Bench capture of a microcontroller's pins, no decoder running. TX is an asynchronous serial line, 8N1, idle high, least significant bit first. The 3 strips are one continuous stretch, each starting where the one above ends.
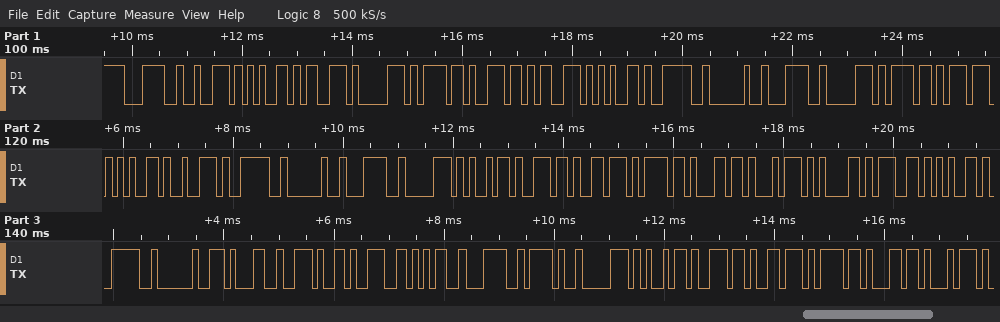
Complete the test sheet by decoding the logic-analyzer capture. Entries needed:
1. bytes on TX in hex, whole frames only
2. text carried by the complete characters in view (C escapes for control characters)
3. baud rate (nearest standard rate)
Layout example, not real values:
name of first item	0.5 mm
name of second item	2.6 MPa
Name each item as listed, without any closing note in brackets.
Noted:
bytes on TX in hex, whole frames only	3C 72 65 73 70 6F 6E 73 65 3E 20 3C 70 6F 77 65 72 3E 20 3C 70 69 6E 76 6F 6C 74 61 67 65 3E 20 31 2E 39 35 3C 2F 70 69 6E 76 6F 6C 74
text carried by the complete characters in view	"<response> <power> <pinvoltage> 1.95</pinvolt"
baud rate	9600 baud
